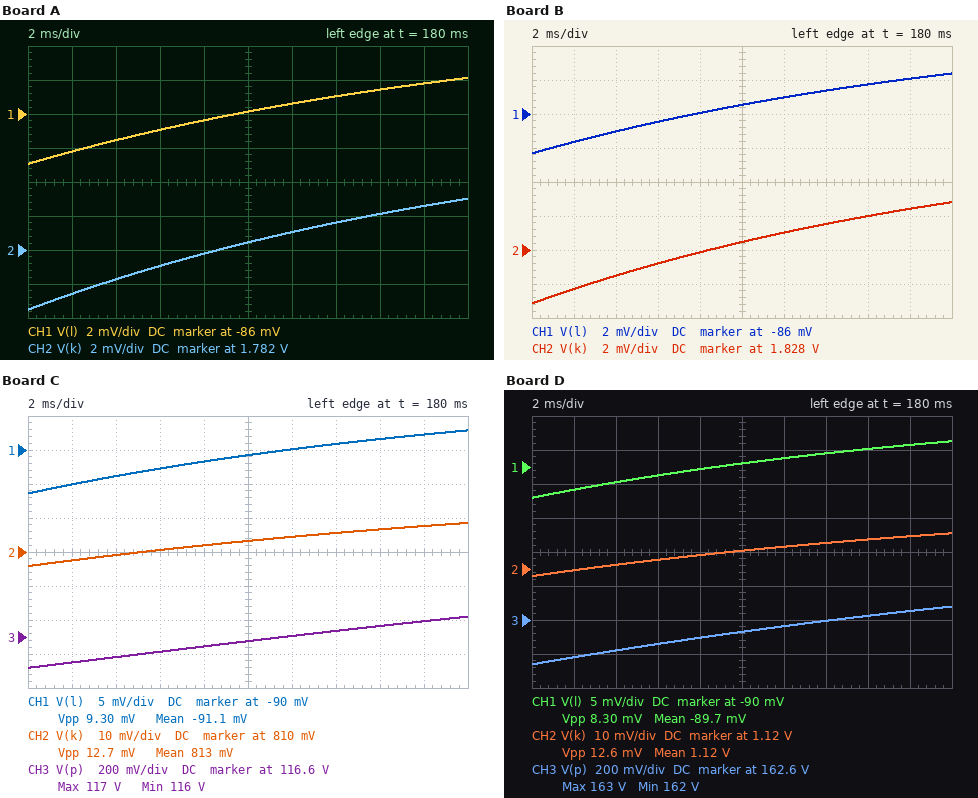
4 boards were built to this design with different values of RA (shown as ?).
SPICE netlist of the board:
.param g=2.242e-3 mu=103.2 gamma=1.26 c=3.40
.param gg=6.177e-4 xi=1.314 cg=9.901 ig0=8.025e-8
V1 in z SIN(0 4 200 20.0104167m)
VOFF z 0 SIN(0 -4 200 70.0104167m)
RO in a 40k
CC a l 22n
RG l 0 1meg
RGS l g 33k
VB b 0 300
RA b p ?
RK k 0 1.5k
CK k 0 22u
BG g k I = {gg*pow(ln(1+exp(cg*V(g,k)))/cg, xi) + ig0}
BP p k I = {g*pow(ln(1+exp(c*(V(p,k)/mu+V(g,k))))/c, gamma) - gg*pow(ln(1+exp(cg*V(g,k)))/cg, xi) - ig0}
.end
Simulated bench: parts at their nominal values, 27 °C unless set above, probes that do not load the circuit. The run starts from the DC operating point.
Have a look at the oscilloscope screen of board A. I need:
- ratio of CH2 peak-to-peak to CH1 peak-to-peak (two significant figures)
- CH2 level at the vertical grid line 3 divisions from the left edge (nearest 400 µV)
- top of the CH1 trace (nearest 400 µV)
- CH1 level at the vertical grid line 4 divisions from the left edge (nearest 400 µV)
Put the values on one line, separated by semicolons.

1.3; 1.7812 V; -84.0 mV; -86.4 mV
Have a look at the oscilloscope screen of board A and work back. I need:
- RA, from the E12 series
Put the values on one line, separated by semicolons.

39 kΩ
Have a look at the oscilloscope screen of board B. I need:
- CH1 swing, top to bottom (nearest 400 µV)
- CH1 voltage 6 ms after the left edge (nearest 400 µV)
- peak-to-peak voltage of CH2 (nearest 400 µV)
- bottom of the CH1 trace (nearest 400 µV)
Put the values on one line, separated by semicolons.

4.8 mV; -86.4 mV; 6.0 mV; -88.4 mV
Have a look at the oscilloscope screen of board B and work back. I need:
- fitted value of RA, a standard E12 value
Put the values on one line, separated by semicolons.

33 kΩ
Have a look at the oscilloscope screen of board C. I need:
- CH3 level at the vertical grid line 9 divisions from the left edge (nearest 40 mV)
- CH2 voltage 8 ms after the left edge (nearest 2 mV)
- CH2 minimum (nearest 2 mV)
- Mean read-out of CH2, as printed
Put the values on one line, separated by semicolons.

116.68 V; 812 mV; 806 mV; 813 mV
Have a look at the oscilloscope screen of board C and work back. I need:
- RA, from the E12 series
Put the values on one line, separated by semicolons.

330 kΩ
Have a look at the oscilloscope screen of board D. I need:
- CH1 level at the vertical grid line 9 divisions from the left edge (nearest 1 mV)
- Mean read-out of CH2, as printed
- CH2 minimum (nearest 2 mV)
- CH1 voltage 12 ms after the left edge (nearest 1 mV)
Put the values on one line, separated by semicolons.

-87 mV; 1.12 V; 1.118 V; -89 mV
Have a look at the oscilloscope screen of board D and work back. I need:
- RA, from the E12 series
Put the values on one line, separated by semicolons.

180 kΩ
